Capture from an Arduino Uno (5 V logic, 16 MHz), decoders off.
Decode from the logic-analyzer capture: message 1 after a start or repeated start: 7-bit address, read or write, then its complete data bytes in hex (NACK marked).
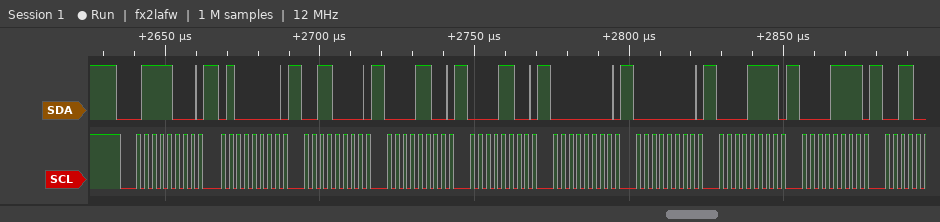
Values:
0x3C write: 40 30 0C 0C 00 00 0F 0F
